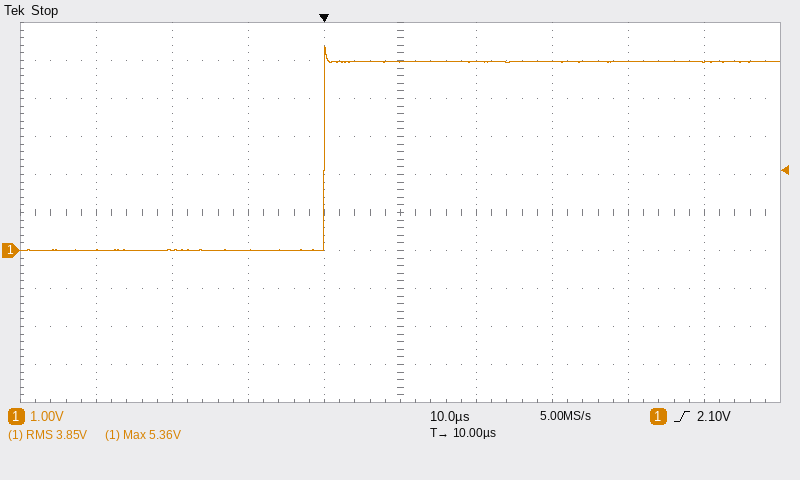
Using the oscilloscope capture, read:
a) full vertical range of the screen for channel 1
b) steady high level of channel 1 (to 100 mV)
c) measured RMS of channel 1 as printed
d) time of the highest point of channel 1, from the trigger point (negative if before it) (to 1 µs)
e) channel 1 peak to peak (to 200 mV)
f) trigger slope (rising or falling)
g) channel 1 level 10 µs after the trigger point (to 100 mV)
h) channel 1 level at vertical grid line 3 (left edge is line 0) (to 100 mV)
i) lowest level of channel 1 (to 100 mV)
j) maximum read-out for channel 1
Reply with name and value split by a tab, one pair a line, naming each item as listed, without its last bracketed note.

full vertical range of the screen for channel 1	10 V
steady high level of channel 1	5.0 V
measured RMS of channel 1 as printed	3.85 V
time of the highest point of channel 1, from the trigger point (negative if before it)	0 µs
channel 1 peak to peak	5.4 V
trigger slope	rising
channel 1 level 10 µs after the trigger point	5.0 V
channel 1 level at vertical grid line 3 (left edge is line 0)	0.0 V
lowest level of channel 1	0.0 V
maximum read-out for channel 1	5.36 V
